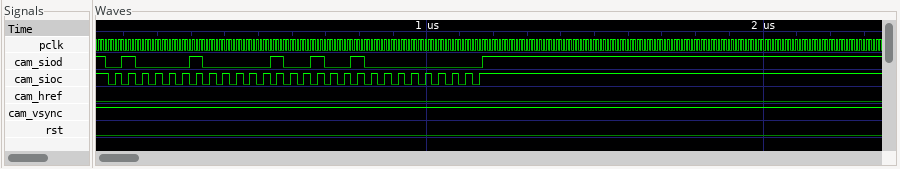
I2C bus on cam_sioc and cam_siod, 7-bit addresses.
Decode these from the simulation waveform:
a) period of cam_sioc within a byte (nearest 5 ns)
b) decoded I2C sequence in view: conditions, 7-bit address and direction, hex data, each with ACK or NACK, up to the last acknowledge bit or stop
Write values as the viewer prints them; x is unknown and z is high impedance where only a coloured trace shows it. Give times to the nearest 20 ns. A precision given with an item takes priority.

40 ns
start, address 21 write ACK, 12 ACK, 80 ACK, stop
